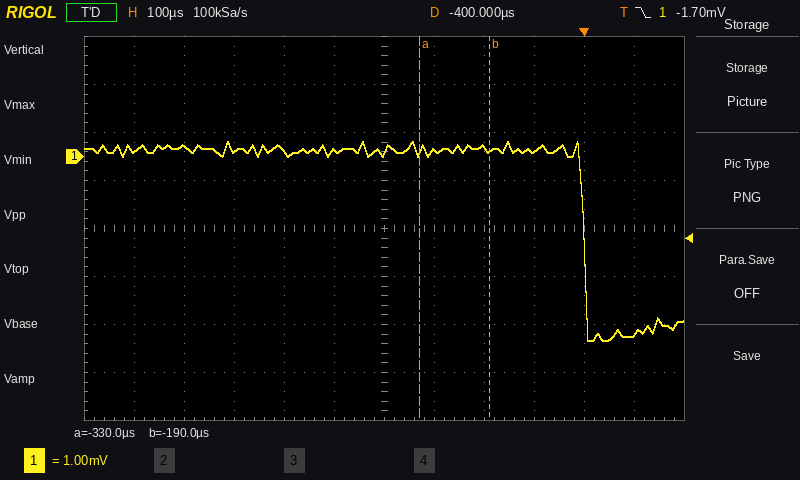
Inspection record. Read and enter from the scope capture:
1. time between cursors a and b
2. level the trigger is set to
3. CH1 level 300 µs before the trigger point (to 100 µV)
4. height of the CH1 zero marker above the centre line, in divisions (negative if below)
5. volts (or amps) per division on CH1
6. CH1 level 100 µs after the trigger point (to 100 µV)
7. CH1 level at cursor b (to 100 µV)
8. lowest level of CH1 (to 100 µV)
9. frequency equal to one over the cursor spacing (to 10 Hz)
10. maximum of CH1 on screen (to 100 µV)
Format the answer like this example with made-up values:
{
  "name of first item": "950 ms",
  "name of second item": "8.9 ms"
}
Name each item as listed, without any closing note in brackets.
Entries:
{
  "time between cursors a and b": "140 µs",
  "level the trigger is set to": "-1.70 mV",
  "CH1 level 300 µs before the trigger point": "100 µV",
  "height of the CH1 zero marker above the centre line, in divisions": "+1.5 div",
  "volts (or amps) per division on CH1": "1 mV",
  "CH1 level 100 µs after the trigger point": "-3.7 mV",
  "CH1 level at cursor b": "100 µV",
  "lowest level of CH1": "-3.8 mV",
  "frequency equal to one over the cursor spacing": "7.14 kHz",
  "maximum of CH1 on screen": "300 µV"
}
